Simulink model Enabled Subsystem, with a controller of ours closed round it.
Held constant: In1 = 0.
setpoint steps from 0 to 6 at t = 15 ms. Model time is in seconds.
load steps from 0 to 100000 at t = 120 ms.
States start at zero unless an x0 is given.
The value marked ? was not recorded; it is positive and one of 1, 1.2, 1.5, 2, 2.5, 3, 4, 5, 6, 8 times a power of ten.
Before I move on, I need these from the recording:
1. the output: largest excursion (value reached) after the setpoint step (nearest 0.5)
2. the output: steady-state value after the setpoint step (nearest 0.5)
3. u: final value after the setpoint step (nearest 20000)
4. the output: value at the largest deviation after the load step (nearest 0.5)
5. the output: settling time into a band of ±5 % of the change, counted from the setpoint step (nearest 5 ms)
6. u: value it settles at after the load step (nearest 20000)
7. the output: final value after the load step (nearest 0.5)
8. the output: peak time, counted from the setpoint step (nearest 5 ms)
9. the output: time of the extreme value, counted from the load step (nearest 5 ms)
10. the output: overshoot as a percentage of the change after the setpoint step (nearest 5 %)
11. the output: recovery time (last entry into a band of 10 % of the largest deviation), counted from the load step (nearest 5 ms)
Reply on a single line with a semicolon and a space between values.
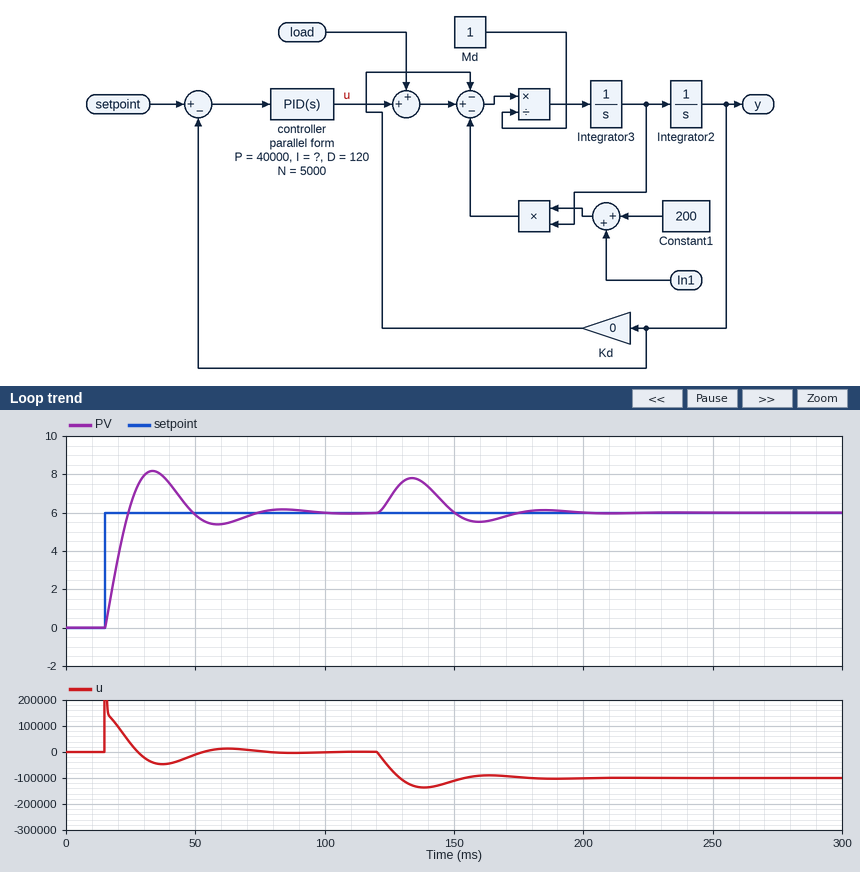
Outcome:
8.0; 6.0; 0; 8.0; 55 ms; -100000; 6.0; 20 ms; 15 ms; 35 %; 50 ms
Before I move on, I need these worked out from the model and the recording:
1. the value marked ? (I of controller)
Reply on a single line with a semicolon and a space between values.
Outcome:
4e+06
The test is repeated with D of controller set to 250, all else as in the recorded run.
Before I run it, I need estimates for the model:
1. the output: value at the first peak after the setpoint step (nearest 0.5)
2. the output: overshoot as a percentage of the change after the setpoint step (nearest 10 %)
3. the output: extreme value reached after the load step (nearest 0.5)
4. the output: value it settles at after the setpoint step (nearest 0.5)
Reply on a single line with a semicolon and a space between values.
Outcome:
7.5; 20 %; 7.5; 6.0
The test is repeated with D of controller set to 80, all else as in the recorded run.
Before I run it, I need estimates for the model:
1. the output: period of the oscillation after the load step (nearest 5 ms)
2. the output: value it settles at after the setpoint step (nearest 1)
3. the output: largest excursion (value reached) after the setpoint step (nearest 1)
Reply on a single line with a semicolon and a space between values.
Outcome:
45 ms; 6; 9
